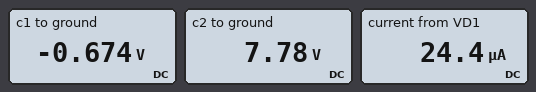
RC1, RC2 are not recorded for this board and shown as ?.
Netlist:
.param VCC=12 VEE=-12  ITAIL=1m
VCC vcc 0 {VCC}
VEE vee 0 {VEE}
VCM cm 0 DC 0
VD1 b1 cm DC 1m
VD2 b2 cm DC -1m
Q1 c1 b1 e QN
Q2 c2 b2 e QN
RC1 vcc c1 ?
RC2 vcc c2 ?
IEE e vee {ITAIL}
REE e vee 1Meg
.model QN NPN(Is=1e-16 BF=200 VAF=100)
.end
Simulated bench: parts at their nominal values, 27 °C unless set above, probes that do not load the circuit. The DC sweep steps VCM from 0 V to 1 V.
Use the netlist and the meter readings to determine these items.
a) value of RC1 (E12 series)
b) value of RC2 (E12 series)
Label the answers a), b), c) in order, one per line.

a) 27 kΩ
b) 8.2 kΩ
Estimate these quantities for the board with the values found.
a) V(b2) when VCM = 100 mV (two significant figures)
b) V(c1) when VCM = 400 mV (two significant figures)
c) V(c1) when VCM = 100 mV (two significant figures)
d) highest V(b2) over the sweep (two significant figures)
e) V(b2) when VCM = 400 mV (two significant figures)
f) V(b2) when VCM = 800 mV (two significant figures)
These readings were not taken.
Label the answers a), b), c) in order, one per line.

a) 99 mV
b) -280 mV
c) -580 mV
d) 1.0 V
e) 400 mV
f) 800 mV
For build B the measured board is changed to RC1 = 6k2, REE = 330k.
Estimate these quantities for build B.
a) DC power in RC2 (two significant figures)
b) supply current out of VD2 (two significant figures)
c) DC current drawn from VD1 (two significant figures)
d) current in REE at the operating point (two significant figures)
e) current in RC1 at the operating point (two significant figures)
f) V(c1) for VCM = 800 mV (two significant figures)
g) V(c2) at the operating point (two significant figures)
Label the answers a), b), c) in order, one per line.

a) 2.0 mW
b) 2.3 µA
c) 2.5 µA
d) 34 µA
e) 540 µA
f) 8.7 V
g) 8.0 V
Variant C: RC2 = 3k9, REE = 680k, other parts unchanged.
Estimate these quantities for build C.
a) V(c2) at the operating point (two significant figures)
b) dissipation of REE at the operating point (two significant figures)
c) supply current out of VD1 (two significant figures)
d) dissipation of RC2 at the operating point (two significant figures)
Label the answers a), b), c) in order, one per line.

a) 10 V
b) 190 µW
c) 23 µA
d) 1.1 mW
